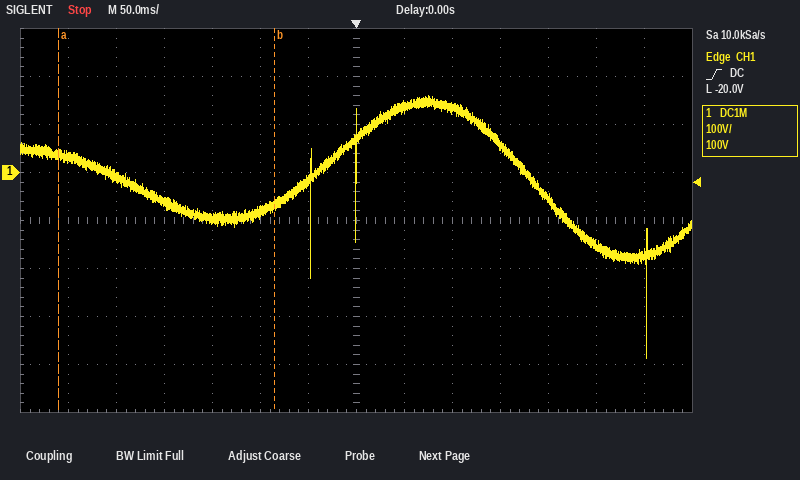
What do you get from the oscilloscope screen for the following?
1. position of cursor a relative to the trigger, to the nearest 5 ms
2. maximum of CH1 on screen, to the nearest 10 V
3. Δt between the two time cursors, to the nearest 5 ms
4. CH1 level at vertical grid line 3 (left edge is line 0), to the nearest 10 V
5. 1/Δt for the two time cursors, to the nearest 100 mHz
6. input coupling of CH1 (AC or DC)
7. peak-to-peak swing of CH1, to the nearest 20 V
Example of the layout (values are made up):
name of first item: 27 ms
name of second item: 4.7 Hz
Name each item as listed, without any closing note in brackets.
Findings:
position of cursor a relative to the trigger, to the nearest 5 ms: -310 ms
maximum of CH1 on screen, to the nearest 10 V: 160 V
Δt between the two time cursors, to the nearest 5 ms: 225 ms
CH1 level at vertical grid line 3 (left edge is line 0), to the nearest 10 V: -60 V
1/Δt for the two time cursors, to the nearest 100 mHz: 4.4 Hz
input coupling of CH1: DC
peak-to-peak swing of CH1, to the nearest 20 V: 540 V
